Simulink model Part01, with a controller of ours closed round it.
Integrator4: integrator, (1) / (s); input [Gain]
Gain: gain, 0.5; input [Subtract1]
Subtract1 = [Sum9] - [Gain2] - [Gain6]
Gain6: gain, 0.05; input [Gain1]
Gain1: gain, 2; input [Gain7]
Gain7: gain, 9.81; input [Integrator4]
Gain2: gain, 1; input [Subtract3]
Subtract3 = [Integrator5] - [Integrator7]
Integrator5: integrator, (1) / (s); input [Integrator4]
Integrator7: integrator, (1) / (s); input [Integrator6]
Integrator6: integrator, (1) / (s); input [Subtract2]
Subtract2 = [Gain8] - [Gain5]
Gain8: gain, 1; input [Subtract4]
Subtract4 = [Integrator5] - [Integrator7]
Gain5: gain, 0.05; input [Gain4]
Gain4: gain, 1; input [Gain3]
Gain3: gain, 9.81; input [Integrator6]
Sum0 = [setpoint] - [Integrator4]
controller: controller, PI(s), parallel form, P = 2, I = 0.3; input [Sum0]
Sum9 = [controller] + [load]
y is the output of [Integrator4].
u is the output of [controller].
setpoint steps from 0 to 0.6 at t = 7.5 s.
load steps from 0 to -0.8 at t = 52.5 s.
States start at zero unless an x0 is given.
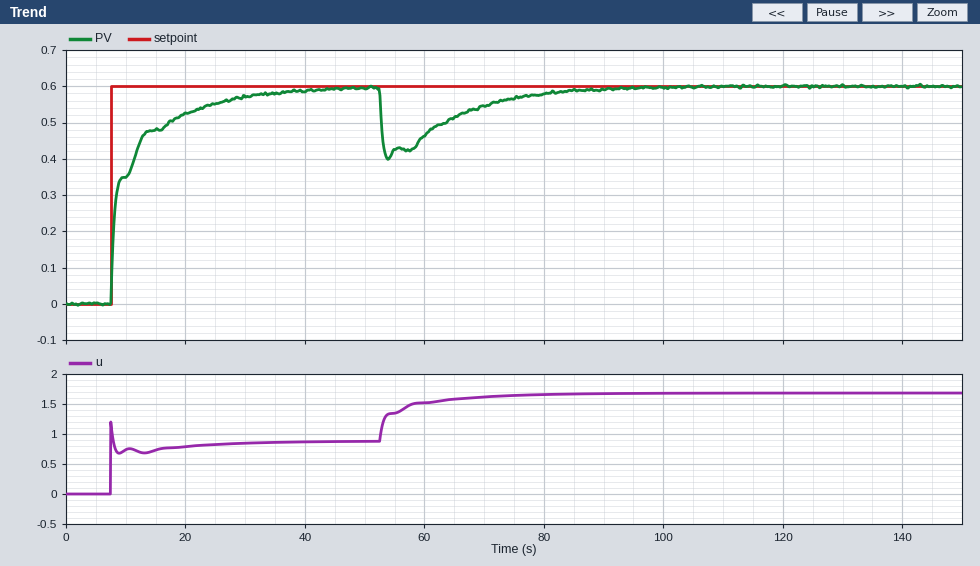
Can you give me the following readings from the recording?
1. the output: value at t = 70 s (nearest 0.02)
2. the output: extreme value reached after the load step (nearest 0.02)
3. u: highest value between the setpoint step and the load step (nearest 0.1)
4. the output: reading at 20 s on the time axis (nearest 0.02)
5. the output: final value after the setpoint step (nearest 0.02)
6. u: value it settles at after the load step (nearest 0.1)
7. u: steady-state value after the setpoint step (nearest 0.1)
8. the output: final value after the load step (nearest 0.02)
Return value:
0.54
0.40
1.2
0.52
0.60
1.7
0.9
0.60
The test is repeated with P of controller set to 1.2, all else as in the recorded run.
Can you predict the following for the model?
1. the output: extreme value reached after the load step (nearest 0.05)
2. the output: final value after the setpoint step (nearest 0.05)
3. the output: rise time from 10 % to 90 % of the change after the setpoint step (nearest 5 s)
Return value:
0.35
0.60
15 s
